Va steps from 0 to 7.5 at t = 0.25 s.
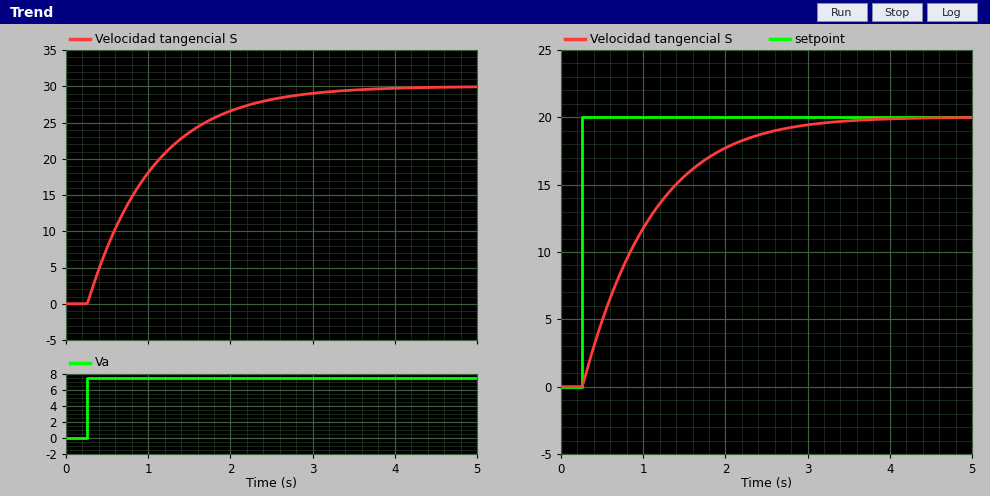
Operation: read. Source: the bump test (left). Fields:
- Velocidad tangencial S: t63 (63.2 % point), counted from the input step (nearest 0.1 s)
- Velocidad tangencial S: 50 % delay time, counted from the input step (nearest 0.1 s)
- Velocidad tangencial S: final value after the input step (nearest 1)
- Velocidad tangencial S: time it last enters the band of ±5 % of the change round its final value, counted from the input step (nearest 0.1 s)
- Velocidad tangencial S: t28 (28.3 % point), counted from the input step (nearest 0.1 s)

0.8 s
0.6 s
30
2.4 s
0.3 s
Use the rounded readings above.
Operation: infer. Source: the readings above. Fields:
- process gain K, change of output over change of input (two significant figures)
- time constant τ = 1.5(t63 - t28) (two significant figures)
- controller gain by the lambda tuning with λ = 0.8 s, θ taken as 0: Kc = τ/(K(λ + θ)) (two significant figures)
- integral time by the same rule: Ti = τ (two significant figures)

4.0
0.75 s
0.23
0.75 s
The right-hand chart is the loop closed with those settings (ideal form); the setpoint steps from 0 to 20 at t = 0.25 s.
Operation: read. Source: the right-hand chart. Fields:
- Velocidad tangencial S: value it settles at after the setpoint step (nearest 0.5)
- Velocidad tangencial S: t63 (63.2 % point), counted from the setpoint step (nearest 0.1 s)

20.0
0.8 s
